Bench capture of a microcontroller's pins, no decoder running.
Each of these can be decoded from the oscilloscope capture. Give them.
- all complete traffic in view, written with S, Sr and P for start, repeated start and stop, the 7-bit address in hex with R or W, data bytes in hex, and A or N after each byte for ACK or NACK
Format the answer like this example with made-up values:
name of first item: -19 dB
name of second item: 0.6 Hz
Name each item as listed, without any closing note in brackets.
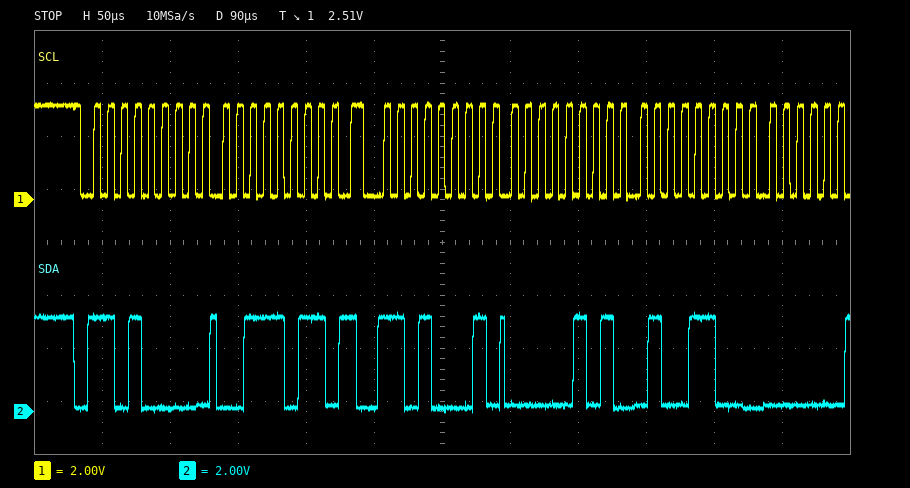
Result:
all complete traffic in view, written with S, Sr and P for start, repeated start and stop, the 7-bit address in hex with R or W, data bytes in hex, and A or N after each byte for ACK or NACK: S 68W A 3B A Sr 68R A 05 A 4C A
